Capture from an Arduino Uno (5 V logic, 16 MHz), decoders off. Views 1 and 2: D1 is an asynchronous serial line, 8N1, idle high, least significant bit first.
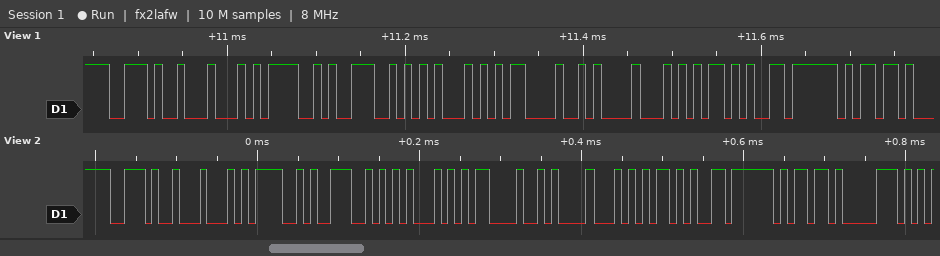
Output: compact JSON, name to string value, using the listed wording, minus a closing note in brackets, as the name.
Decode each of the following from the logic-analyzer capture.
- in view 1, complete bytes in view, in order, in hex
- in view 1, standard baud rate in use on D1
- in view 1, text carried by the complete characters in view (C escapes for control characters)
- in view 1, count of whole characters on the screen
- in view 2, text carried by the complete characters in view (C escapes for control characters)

{"in view 1, complete bytes in view, in order, in hex": "2E 44 4F 4E 45 0D 0A 54 65 6D", "in view 1, standard baud rate in use on D1": "115200 baud", "in view 1, text carried by the complete characters in view": "\".DONE\\r\\nTem\"", "in view 1, count of whole characters on the screen": "10", "in view 2, text carried by the complete characters in view": "\".DONE\\r\\nTemp\""}
